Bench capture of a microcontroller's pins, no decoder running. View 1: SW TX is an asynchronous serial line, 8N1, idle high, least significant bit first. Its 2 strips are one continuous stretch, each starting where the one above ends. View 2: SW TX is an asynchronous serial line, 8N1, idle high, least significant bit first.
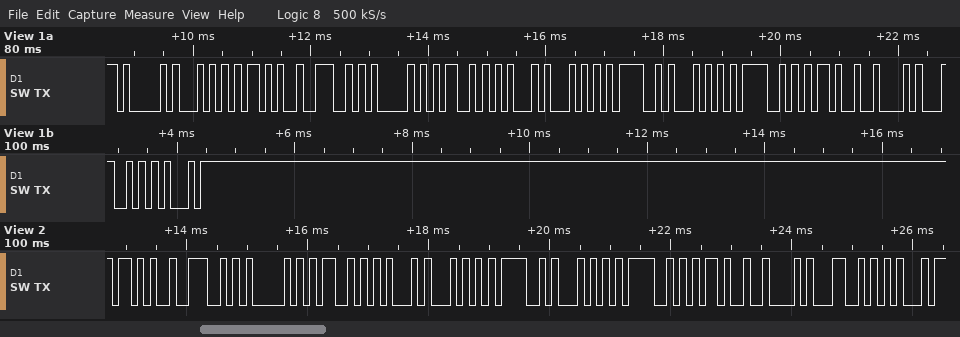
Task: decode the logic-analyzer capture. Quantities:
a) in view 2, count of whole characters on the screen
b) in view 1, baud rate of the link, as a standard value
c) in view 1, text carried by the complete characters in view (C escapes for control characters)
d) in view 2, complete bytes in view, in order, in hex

13
9600 baud
"AT+NAMETOTO-BLE"
2B 4E 41 4D 45 54 4F 54 4F 2D 42 4C 45
